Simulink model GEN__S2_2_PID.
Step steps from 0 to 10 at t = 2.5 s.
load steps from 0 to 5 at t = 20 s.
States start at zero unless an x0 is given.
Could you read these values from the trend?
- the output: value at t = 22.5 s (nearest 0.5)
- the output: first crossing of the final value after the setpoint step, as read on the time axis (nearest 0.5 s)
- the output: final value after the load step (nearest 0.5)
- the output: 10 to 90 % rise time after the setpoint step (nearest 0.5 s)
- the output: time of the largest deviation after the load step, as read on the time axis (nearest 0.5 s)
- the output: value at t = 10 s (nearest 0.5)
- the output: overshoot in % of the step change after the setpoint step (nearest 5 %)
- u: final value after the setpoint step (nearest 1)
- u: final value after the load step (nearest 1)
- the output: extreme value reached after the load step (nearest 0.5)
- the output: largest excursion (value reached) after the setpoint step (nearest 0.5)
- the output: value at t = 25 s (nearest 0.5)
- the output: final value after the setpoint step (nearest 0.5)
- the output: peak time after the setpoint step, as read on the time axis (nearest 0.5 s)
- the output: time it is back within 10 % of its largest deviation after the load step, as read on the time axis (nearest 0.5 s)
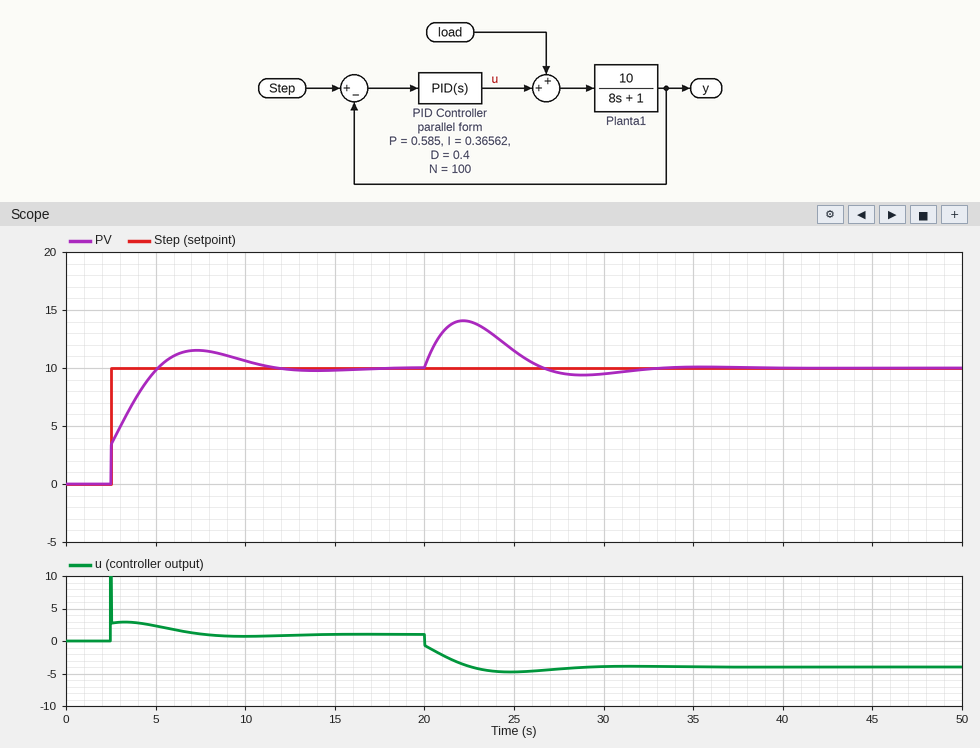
14.0
5.0 s
10.0
2.0 s
22.0 s
10.5
15 %
1
-4
14.0
11.5
11.5
10.0
7.5 s
30.5 s
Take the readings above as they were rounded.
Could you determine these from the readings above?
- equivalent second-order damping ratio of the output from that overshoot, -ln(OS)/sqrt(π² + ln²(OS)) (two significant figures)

0.52
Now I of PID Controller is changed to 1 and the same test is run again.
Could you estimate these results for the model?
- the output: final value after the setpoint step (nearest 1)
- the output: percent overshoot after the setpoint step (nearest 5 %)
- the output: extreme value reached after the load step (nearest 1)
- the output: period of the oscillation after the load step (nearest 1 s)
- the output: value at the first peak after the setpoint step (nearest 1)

10
25 %
13
7 s
13
